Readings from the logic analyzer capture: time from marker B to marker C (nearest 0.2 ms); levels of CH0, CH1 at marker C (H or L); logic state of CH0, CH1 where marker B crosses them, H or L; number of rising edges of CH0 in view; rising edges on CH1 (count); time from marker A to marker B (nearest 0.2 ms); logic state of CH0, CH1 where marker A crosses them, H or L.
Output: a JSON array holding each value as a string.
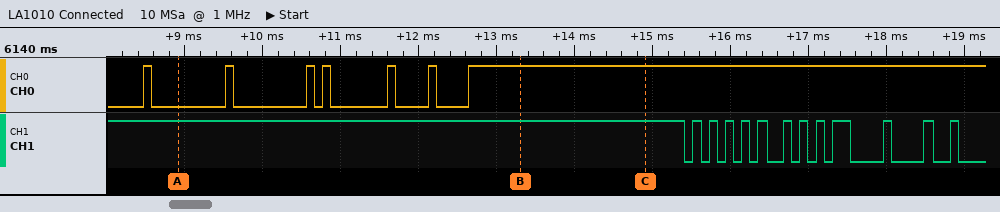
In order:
["1.6 ms", "CH0=H, CH1=H", "CH0=H, CH1=H", "7", "12", "4.4 ms", "CH0=L, CH1=H"]
